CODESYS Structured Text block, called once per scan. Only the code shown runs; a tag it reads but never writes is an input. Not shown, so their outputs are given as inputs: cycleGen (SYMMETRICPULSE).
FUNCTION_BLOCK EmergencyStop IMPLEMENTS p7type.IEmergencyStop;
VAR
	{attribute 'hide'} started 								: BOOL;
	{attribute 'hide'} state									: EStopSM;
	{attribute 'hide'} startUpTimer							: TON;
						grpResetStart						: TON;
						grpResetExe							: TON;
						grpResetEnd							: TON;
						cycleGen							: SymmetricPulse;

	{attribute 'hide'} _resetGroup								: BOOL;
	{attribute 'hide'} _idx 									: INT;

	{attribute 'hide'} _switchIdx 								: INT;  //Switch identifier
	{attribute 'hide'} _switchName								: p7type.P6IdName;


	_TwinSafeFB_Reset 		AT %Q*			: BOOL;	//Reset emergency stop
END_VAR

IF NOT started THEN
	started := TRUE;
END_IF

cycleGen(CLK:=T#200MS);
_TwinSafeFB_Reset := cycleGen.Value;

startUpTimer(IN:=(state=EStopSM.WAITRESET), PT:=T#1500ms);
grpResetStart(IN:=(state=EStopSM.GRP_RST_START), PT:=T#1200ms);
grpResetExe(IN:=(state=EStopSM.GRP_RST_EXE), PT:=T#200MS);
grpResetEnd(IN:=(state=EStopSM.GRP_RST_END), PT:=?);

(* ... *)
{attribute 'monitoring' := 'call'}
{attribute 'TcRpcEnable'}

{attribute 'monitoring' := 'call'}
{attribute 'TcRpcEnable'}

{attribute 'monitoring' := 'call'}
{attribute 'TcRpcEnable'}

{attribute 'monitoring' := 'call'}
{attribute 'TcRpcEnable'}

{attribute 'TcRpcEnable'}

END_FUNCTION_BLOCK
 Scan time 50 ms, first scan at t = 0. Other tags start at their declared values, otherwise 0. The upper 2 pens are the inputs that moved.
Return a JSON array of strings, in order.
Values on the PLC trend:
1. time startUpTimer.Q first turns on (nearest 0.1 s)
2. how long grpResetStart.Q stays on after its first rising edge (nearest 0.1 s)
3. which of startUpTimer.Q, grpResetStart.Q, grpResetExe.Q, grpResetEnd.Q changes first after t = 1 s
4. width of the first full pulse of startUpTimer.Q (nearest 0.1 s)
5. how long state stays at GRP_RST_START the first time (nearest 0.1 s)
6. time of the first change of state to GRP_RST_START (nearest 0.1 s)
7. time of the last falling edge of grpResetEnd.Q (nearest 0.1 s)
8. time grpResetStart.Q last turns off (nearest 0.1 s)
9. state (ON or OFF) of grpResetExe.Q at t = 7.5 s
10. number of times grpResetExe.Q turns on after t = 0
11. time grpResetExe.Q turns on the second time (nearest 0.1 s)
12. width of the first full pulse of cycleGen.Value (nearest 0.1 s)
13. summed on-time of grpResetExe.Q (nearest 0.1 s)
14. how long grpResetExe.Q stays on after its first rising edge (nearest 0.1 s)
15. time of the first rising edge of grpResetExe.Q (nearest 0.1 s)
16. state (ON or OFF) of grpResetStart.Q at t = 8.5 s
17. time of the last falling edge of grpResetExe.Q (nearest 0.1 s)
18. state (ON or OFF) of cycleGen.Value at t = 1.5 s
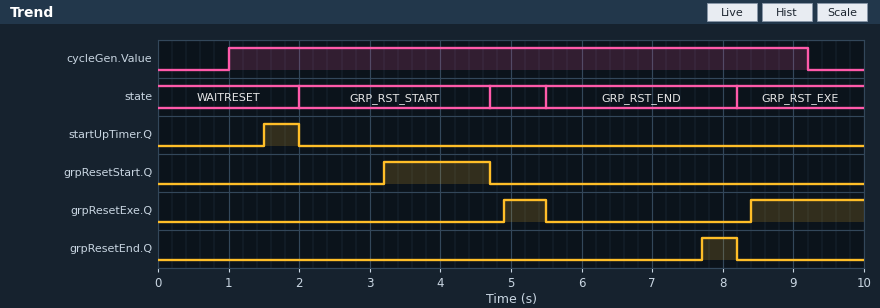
["1.5 s", "1.5 s", "startUpTimer.Q", "0.5 s", "2.7 s", "2.0 s", "8.2 s", "4.7 s", "OFF", "2", "8.4 s", "8.2 s", "2.2 s", "0.6 s", "4.9 s", "OFF", "5.5 s", "ON"]
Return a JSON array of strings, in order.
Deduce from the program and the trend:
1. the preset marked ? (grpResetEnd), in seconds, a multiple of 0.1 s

["2.2 s"]
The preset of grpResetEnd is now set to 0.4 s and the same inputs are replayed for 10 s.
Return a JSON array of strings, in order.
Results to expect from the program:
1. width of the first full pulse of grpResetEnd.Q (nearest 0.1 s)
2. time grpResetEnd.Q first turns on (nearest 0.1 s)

["2.3 s", "5.9 s"]
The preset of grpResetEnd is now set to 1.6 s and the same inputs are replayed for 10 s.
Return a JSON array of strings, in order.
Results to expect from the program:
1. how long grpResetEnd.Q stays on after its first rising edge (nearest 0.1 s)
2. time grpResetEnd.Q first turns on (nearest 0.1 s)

["1.1 s", "7.1 s"]
